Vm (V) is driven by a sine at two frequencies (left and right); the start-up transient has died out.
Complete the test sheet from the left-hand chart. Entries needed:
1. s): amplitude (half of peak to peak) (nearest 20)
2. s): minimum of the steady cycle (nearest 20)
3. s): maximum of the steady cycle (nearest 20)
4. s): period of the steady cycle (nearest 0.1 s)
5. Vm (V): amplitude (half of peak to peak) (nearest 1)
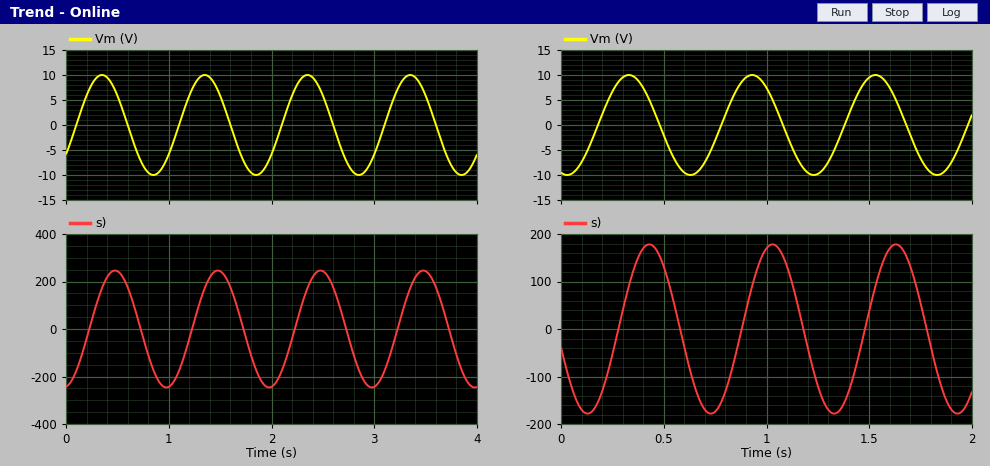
240
-240
240
1.0 s
10
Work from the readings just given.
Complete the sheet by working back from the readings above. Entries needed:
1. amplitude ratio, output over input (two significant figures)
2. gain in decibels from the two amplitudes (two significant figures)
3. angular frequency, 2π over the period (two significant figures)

24
28 dB
6.3 rad/s
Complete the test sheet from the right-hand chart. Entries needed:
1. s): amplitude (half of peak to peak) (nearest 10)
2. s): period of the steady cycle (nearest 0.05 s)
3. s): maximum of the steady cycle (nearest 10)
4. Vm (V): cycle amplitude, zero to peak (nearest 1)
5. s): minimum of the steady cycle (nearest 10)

180
0.60 s
180
10
-180
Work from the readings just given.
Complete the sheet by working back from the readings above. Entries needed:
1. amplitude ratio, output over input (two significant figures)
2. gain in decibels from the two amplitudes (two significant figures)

18
25 dB
